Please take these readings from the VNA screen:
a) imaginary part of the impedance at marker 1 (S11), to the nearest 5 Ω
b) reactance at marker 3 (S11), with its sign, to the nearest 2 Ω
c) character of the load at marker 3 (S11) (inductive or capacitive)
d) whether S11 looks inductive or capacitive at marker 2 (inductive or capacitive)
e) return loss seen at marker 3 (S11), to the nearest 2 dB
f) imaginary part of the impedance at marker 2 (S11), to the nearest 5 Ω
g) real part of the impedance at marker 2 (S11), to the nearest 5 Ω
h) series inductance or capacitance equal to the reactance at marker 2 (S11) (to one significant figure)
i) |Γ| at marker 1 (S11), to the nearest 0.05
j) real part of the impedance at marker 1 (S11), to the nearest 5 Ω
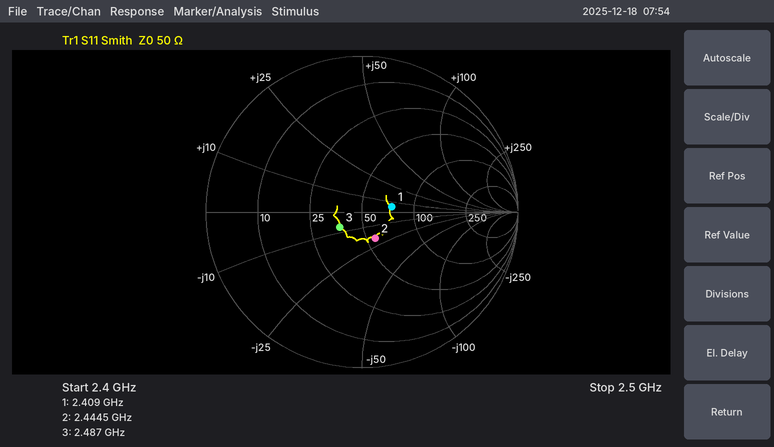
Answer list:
+5 Ω
-8 Ω
capacitive
capacitive
16 dB
-20 Ω
55 Ω
3 pF
0.20
75 Ω
